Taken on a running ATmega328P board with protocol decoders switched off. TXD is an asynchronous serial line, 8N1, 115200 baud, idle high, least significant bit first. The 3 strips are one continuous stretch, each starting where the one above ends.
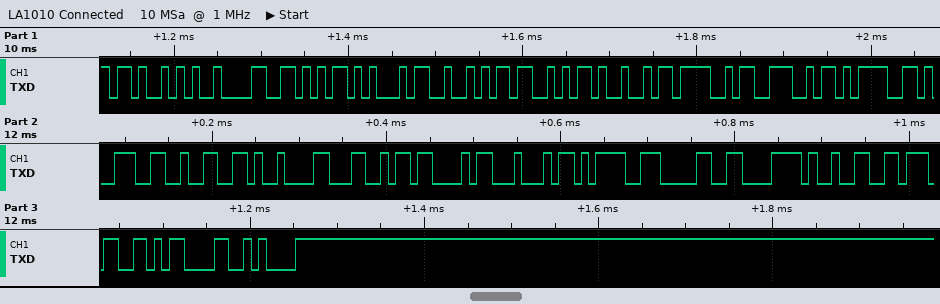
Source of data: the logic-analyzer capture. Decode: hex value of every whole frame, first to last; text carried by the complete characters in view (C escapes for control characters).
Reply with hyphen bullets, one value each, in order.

- 0x4B 0x09 0x56 0x45 0x52 0x53 0x49 0x4F 0x4E 0x3D 0x39 0x32 0x09 0x4C 0x43 0x44 0x3D 0x30 0x78 0x32 0x37 0x0D 0x0A
- "K\tVERSION=92\tLCD=0x27\r\n"
